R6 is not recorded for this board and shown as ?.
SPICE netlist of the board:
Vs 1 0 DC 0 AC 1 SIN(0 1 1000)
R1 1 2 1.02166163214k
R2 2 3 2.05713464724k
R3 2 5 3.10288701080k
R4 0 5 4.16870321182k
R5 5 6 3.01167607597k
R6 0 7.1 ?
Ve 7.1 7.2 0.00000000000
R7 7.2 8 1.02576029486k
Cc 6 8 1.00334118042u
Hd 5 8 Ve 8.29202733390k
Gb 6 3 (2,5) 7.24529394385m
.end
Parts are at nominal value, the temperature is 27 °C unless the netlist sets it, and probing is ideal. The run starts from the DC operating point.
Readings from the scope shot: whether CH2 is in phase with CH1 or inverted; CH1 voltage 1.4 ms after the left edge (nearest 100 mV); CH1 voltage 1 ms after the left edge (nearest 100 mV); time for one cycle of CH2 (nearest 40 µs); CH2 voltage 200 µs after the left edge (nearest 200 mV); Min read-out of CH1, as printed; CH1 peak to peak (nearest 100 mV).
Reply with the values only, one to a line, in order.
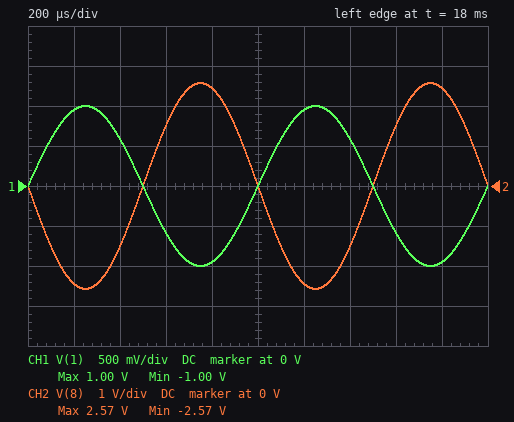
inverted
600 mV
0 V
1.00 ms
-2.4 V
-1.00 V
2.0 V
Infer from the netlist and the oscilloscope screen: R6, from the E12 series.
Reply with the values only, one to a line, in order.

4.7 kΩ
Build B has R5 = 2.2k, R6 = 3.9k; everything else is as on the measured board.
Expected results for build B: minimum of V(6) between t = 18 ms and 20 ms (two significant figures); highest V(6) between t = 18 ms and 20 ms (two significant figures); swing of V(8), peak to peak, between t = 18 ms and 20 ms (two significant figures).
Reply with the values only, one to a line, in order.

-1.5 V
1.5 V
3.1 V
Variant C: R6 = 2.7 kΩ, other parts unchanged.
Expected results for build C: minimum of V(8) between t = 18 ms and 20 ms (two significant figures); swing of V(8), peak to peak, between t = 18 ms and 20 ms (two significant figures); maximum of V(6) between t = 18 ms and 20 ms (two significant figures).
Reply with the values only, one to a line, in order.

-800 mV
1.6 V
800 mV
